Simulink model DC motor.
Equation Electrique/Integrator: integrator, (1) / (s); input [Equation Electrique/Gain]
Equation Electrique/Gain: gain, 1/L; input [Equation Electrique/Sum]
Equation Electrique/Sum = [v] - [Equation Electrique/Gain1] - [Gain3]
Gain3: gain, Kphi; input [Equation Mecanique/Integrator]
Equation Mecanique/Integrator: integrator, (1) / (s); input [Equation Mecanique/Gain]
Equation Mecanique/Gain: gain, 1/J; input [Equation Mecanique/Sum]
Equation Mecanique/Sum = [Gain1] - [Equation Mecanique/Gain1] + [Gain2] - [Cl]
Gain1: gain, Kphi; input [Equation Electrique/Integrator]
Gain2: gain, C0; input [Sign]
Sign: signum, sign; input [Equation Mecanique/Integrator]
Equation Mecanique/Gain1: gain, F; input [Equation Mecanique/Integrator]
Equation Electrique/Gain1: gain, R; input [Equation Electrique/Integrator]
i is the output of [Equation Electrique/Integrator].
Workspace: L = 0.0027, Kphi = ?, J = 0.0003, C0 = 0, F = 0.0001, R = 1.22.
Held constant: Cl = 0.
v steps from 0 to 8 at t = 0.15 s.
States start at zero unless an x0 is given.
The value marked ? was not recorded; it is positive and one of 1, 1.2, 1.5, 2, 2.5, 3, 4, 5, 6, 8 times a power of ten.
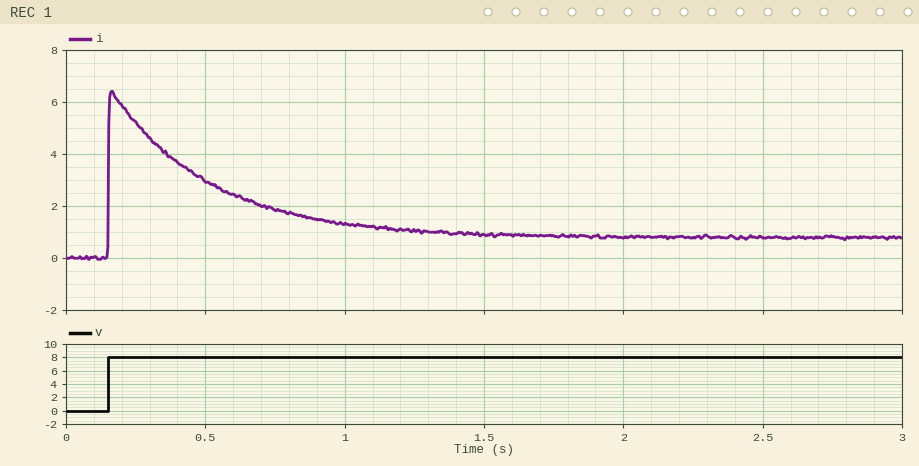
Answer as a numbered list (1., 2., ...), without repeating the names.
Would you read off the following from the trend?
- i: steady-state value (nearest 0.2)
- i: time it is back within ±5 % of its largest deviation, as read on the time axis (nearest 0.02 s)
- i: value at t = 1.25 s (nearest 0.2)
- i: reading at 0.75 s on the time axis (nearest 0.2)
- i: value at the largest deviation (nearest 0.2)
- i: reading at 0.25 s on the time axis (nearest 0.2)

1. 0.8
2. 1.18 s
3. 1.0
4. 1.8
5. 6.4
6. 5.2
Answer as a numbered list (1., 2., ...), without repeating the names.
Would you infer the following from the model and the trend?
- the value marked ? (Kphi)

1. 0.03
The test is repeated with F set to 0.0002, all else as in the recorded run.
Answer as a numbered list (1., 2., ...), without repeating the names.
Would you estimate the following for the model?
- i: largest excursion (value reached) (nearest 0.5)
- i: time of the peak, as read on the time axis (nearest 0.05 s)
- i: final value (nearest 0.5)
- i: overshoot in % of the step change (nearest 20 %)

1. 6.5
2. 0.15 s
3. 1.5
4. 360 %
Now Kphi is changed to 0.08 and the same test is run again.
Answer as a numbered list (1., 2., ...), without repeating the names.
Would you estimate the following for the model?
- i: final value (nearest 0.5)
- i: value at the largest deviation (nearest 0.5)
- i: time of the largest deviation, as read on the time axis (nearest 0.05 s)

1. 0.0
2. 6.0
3. 0.15 s
